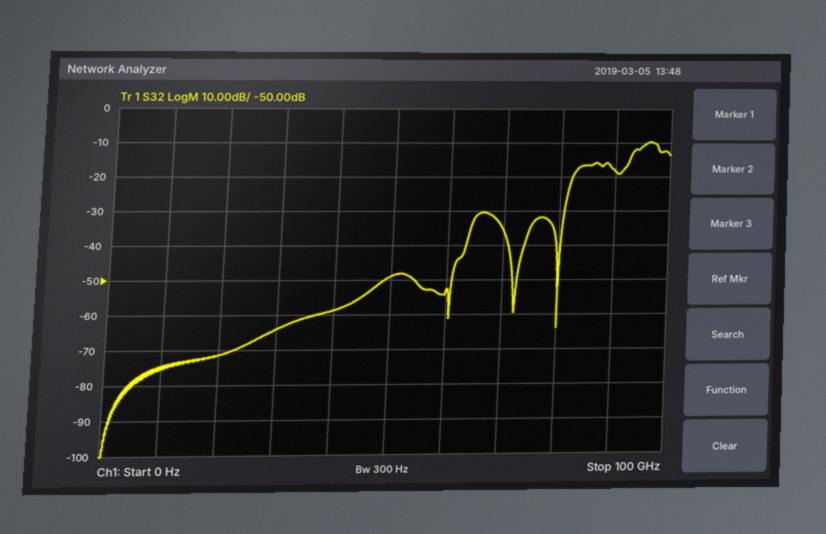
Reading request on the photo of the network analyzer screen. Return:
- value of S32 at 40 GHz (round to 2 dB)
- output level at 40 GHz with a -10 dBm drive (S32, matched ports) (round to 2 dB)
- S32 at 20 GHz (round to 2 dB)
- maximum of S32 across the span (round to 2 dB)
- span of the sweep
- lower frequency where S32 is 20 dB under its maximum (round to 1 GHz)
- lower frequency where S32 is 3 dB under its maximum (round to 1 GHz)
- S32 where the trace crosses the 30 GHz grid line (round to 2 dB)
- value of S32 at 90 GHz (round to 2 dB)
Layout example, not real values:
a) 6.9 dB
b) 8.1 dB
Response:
a) -58 dB
b) -68 dBm
c) -72 dB
d) -10 dB
e) 100 GHz
f) 81 GHz
g) 93 GHz
h) -64 dB
i) -18 dB
